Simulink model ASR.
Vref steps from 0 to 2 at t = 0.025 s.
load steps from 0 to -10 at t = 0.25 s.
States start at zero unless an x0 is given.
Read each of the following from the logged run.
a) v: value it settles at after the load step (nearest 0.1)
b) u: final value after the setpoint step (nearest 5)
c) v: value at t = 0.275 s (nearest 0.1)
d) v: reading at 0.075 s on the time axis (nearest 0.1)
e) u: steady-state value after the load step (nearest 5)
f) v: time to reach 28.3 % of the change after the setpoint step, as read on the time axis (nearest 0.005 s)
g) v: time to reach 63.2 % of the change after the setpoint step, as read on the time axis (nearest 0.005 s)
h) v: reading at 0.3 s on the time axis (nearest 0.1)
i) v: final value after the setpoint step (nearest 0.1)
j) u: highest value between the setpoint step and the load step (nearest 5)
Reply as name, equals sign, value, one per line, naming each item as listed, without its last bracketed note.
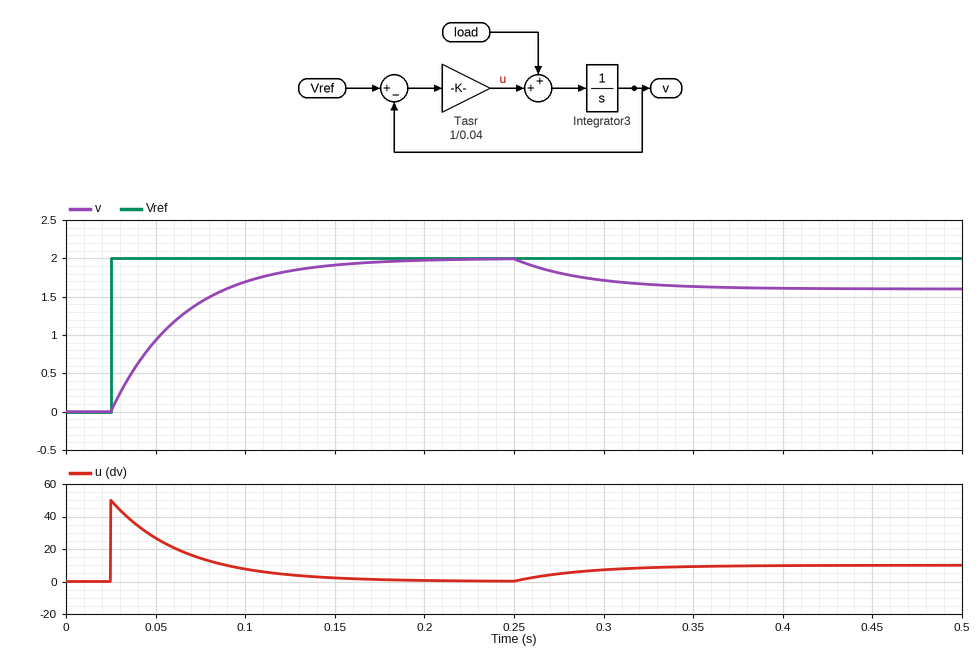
v: value it settles at after the load step = 1.6
u: final value after the setpoint step = 0
v: value at t = 0.275 s = 1.8
v: reading at 0.075 s on the time axis = 1.4
u: steady-state value after the load step = 10
v: time to reach 28.3 % of the change after the setpoint step, as read on the time axis = 0.040 s
v: time to reach 63.2 % of the change after the setpoint step, as read on the time axis = 0.065 s
v: reading at 0.3 s on the time axis = 1.7
v: final value after the setpoint step = 2.0
u: highest value between the setpoint step and the load step = 50
